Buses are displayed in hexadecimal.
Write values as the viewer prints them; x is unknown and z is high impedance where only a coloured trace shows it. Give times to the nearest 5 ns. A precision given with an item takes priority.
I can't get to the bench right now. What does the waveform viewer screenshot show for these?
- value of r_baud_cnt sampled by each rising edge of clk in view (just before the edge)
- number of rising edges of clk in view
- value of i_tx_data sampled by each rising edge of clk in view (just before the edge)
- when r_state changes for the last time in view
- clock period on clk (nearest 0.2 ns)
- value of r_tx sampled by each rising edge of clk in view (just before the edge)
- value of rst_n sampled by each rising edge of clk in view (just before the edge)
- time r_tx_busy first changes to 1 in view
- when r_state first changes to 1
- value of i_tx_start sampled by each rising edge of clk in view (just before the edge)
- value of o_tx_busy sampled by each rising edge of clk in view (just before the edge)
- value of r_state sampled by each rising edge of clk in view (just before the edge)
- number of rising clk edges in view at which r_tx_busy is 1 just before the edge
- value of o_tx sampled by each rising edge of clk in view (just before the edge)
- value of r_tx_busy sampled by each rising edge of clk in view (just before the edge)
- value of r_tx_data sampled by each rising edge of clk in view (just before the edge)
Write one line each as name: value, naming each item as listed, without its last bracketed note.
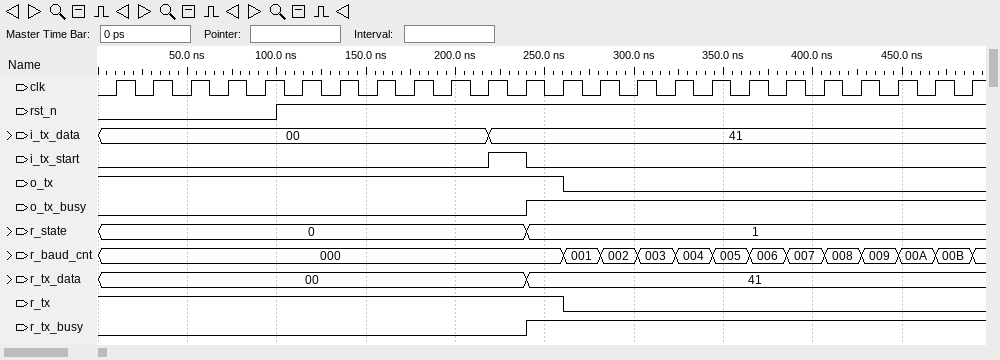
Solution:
value of r_baud_cnt sampled by each rising edge of clk in view: 000, 000, 000, 000, 000, 000, 000, 000, 000, 000, 000, 000, 000, 001, 002, 003, 004, 005, 006, 007, 008, 009, 00A, 00B
number of rising edges of clk in view: 24
value of i_tx_data sampled by each rising edge of clk in view: 00, 00, 00, 00, 00, 00, 00, 00, 00, 00, 00, 41, 41, 41, 41, 41, 41, 41, 41, 41, 41, 41, 41, 41
when r_state changes for the last time in view: 240 ns
clock period on clk: 20.8 ns
value of r_tx sampled by each rising edge of clk in view: 1 1 1 1 1 1 1 1 1 1 1 1 1 0 0 0 0 0 0 0 0 0 0 0
value of rst_n sampled by each rising edge of clk in view: 0 0 0 0 0 1 1 1 1 1 1 1 1 1 1 1 1 1 1 1 1 1 1 1
time r_tx_busy first changes to 1 in view: 240 ns
when r_state first changes to 1: 240 ns
value of i_tx_start sampled by each rising edge of clk in view: 0 0 0 0 0 0 0 0 0 0 0 1 0 0 0 0 0 0 0 0 0 0 0 0
value of o_tx_busy sampled by each rising edge of clk in view: 0 0 0 0 0 0 0 0 0 0 0 0 1 1 1 1 1 1 1 1 1 1 1 1
value of r_state sampled by each rising edge of clk in view: 0, 0, 0, 0, 0, 0, 0, 0, 0, 0, 0, 0, 1, 1, 1, 1, 1, 1, 1, 1, 1, 1, 1, 1
number of rising clk edges in view at which r_tx_busy is 1 just before the edge: 12
value of o_tx sampled by each rising edge of clk in view: 1 1 1 1 1 1 1 1 1 1 1 1 1 0 0 0 0 0 0 0 0 0 0 0
value of r_tx_busy sampled by each rising edge of clk in view: 0 0 0 0 0 0 0 0 0 0 0 0 1 1 1 1 1 1 1 1 1 1 1 1
value of r_tx_data sampled by each rising edge of clk in view: 00, 00, 00, 00, 00, 00, 00, 00, 00, 00, 00, 00, 41, 41, 41, 41, 41, 41, 41, 41, 41, 41, 41, 41
